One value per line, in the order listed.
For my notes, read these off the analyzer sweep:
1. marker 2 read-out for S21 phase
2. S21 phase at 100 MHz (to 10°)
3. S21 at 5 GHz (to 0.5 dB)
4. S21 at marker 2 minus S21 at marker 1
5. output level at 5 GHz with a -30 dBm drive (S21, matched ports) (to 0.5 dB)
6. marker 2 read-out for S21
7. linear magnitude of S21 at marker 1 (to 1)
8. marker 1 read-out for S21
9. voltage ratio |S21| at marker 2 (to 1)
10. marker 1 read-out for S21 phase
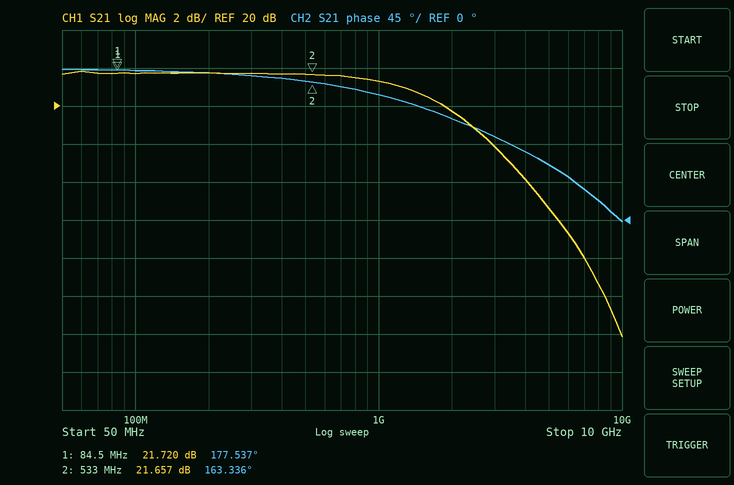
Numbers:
163.336°
180°
14.5 dB
-0.063 dB
-15.5 dBm
21.657 dB
12
21.720 dB
12
177.537°
